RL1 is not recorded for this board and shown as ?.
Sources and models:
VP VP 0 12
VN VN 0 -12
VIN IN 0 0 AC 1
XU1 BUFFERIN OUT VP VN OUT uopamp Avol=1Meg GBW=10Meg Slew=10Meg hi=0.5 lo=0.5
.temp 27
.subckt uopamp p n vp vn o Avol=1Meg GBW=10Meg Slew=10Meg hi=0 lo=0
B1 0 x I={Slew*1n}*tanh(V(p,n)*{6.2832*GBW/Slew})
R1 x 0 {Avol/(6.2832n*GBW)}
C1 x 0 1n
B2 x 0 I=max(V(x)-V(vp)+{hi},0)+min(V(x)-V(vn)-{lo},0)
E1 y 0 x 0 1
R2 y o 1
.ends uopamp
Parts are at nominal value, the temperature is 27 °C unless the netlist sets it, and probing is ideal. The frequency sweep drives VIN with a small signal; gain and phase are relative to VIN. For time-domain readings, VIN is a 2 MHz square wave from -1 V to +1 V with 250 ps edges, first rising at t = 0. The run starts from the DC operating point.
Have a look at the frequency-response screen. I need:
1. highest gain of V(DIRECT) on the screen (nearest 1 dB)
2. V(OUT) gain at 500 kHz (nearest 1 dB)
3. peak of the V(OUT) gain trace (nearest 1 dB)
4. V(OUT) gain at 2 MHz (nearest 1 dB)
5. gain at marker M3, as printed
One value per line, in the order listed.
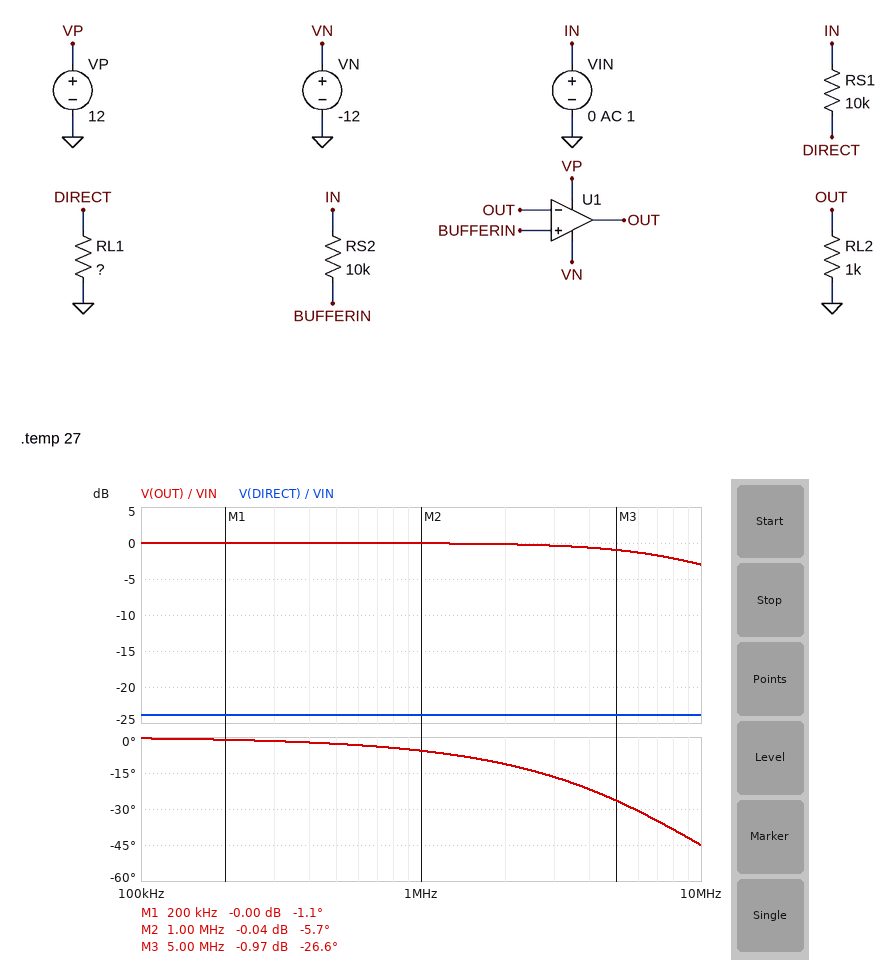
-24 dB
0 dB
0 dB
0 dB
-0.97 dB
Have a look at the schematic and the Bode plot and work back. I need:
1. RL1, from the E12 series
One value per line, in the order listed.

680 Ω
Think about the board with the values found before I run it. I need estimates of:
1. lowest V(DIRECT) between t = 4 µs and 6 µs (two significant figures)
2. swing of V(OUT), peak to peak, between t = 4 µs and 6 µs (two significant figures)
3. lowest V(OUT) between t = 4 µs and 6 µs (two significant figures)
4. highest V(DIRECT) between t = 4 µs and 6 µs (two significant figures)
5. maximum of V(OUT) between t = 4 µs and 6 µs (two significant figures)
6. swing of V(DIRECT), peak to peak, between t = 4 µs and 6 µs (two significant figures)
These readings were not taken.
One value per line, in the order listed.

-64 mV
2.0 V
-1.0 V
64 mV
1.0 V
130 mV
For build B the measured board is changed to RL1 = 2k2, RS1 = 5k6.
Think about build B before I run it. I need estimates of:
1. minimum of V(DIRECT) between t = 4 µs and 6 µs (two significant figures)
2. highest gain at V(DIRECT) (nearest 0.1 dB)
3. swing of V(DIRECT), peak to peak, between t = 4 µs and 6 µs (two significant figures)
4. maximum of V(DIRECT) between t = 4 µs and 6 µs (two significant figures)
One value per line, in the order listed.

-280 mV
-11.0 dB
560 mV
280 mV
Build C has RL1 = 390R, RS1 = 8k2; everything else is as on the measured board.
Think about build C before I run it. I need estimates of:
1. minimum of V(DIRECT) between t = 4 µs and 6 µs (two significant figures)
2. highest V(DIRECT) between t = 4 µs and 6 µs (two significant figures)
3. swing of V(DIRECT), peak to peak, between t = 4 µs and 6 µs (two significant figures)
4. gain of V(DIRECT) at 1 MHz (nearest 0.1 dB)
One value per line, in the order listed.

-45 mV
45 mV
91 mV
-26.9 dB
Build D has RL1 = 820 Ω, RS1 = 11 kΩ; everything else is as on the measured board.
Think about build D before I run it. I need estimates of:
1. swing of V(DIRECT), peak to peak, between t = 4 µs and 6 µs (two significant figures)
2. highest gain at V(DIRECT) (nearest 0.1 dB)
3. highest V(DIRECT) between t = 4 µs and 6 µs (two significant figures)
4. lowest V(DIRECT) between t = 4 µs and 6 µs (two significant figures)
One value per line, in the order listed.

140 mV
-23.2 dB
69 mV
-69 mV
